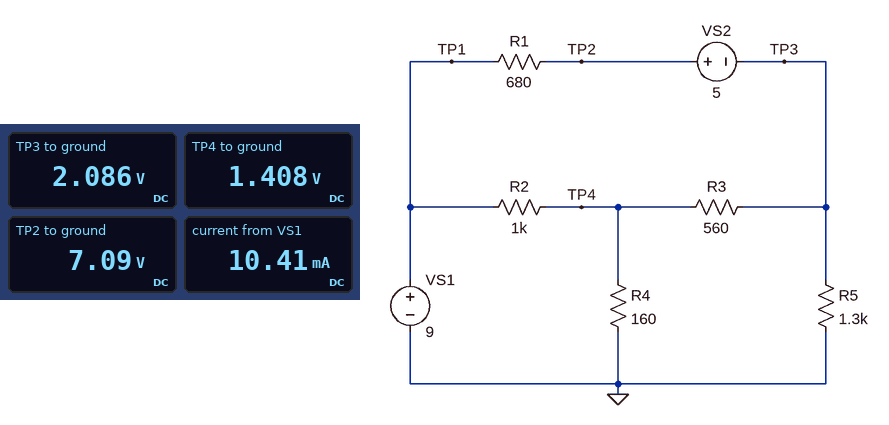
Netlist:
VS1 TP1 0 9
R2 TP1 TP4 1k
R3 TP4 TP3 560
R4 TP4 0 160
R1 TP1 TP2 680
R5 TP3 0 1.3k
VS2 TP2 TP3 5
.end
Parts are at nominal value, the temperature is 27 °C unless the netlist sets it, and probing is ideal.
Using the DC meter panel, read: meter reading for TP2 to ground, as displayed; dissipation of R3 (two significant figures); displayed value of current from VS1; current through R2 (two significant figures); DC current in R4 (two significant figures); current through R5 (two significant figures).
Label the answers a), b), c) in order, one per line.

a) 7.09 V
b) 820 µW
c) 10.41 mA
d) 7.6 mA
e) 8.8 mA
f) 1.6 mA
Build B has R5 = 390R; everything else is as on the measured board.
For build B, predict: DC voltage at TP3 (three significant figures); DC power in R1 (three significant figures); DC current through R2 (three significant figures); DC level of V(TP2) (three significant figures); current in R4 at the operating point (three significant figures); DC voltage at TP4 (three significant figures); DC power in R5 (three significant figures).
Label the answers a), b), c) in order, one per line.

a) 1.40 V
b) 9.93 mW
c) 7.73 mA
d) 6.40 V
e) 7.96 mA
f) 1.27 V
g) 5.03 mW
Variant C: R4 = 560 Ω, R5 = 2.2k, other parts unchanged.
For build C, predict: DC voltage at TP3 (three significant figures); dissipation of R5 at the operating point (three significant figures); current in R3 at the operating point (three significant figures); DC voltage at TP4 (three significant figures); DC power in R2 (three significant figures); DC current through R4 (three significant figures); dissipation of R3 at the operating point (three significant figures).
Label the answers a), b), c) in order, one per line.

a) 3.12 V
b) 4.42 mW
c) 122 µA
d) 3.19 V
e) 33.8 mW
f) 5.69 mA
g) 8.31 µW
